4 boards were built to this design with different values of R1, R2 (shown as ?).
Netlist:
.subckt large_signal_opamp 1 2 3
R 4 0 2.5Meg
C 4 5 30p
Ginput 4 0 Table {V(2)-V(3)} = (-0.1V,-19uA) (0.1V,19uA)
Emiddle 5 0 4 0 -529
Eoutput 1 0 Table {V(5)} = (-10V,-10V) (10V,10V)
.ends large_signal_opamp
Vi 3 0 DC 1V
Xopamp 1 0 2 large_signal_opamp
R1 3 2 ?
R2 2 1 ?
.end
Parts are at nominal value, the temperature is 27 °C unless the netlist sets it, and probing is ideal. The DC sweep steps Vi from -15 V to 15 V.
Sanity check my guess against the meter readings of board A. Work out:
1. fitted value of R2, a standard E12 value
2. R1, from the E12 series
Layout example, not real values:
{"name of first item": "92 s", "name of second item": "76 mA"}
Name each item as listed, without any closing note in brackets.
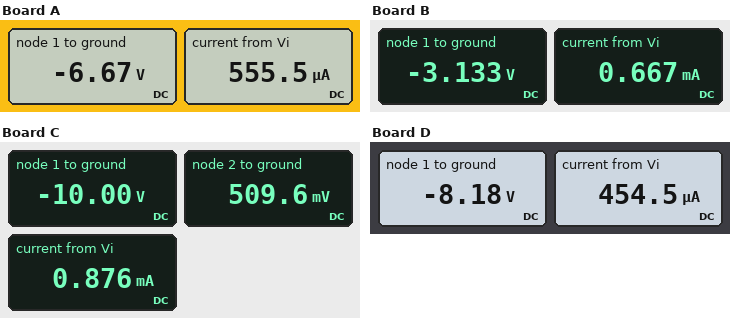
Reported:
{"fitted value of R2, a standard E12 value": "12 kΩ", "R1, from the E12 series": "1.8 kΩ"}
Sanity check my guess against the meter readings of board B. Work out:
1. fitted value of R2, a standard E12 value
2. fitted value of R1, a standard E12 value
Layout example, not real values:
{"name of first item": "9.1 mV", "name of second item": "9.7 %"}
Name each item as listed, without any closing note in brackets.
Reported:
{"fitted value of R2, a standard E12 value": "4.7 kΩ", "fitted value of R1, a standard E12 value": "1.5 kΩ"}
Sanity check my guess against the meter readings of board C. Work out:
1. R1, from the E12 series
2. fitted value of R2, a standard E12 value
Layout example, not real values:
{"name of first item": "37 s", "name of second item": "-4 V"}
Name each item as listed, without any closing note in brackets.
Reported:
{"R1, from the E12 series": "560 Ω", "fitted value of R2, a standard E12 value": "12 kΩ"}
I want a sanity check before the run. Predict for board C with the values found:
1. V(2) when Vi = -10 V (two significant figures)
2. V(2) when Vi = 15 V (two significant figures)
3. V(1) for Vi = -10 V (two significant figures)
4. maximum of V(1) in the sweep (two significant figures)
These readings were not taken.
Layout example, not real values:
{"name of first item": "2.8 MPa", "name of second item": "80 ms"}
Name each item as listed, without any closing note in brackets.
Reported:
{"V(2) when Vi = -10 V": "-9.1 V", "V(2) when Vi = 15 V": "14 V", "V(1) for Vi = -10 V": "10 V", "maximum of V(1) in the sweep": "10 V"}
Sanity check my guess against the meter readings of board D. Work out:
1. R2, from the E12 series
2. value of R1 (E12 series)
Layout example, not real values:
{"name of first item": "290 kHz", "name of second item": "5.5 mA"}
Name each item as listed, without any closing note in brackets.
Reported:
{"R2, from the E12 series": "18 kΩ", "value of R1": "2.2 kΩ"}
